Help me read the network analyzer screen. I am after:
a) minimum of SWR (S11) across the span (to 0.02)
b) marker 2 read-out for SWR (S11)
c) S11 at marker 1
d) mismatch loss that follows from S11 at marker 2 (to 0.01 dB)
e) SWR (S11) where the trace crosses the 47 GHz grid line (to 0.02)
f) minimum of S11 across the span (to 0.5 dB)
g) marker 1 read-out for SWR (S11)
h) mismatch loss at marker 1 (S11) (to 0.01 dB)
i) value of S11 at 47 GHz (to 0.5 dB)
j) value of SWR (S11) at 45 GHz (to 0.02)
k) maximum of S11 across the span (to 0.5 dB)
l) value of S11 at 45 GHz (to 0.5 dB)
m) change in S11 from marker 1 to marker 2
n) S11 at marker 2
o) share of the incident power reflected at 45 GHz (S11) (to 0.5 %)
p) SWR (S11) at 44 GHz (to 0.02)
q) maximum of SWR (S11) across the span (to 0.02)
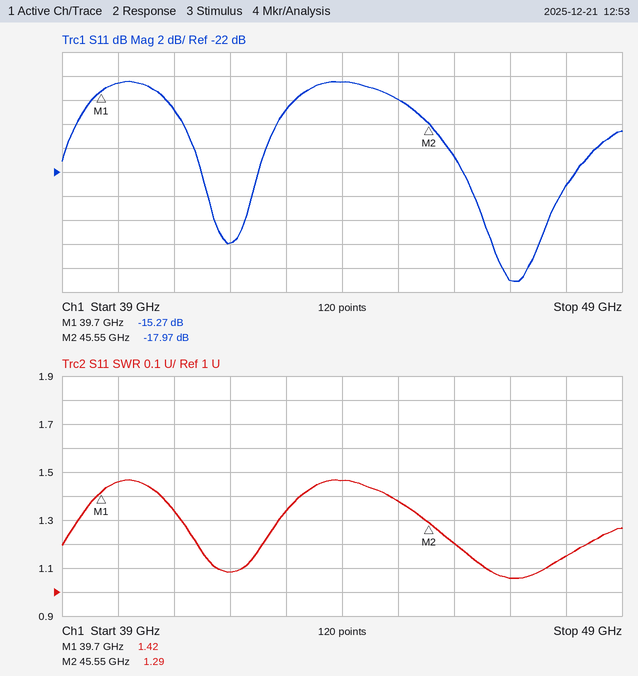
1.06
1.29
-15.27 dB
0.07 dB
1.06
-31.0 dB
1.42
0.13 dB
-31.0 dB
1.38
-14.5 dB
-16.0 dB
-2.70 dB
-17.97 dB
2.5 %
1.46
1.46
